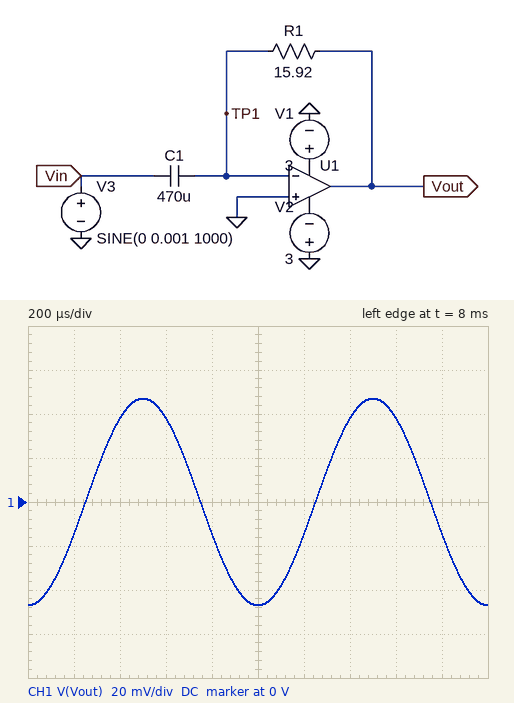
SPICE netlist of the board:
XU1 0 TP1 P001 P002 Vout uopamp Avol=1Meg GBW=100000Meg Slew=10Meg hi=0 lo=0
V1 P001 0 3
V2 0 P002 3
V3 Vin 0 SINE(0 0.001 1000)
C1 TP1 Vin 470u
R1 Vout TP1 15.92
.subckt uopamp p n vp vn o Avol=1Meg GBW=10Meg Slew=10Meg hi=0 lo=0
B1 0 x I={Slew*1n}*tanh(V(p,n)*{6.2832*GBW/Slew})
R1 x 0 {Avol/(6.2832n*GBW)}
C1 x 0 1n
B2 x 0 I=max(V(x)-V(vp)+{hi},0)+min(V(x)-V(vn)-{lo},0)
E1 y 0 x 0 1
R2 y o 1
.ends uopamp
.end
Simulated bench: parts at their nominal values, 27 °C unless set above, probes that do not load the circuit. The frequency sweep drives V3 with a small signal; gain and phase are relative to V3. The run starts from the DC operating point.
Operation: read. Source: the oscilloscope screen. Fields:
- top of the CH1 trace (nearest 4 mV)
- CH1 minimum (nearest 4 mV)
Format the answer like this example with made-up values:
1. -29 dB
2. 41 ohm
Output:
1. 48 mV
2. -48 mV
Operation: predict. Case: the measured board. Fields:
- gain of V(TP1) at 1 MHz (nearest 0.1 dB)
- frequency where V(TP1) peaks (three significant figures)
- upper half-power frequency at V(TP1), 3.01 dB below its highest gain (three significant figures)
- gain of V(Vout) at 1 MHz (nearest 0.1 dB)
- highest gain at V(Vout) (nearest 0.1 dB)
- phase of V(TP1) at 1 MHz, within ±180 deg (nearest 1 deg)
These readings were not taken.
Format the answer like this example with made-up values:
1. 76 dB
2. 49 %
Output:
1. 0 dB
2. 1.42 MHz
3. 1.47 MHz
4. 99.4 dB
5. 119.5 dB
6. 169 deg
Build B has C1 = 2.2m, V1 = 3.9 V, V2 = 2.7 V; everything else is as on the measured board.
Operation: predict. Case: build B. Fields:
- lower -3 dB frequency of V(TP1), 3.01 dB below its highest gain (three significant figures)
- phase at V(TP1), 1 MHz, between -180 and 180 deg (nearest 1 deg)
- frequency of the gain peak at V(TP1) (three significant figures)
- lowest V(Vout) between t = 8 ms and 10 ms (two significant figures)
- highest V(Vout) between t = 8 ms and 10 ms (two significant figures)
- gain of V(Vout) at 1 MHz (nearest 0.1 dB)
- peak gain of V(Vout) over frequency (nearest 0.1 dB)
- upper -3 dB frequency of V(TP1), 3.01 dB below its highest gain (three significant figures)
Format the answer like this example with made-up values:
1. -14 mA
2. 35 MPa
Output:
1. 612 kHz
2. 4 deg
3. 658 kHz
4. -220 mV
5. 220 mV
6. 104.2 dB
7. 119.5 dB
8. 715 kHz
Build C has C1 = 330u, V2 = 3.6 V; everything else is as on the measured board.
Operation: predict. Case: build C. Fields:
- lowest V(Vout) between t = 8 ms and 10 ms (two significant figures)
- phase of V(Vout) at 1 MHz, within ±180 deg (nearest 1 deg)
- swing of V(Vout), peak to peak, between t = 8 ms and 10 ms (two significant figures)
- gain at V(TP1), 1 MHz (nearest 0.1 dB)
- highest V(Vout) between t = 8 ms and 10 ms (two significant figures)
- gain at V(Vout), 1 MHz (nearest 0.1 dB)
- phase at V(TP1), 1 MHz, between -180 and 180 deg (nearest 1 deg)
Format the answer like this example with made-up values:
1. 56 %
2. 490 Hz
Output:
1. -33 mV
2. -93 deg
3. 66 mV
4. -5.3 dB
5. 33 mV
6. 94.1 dB
7. 171 deg
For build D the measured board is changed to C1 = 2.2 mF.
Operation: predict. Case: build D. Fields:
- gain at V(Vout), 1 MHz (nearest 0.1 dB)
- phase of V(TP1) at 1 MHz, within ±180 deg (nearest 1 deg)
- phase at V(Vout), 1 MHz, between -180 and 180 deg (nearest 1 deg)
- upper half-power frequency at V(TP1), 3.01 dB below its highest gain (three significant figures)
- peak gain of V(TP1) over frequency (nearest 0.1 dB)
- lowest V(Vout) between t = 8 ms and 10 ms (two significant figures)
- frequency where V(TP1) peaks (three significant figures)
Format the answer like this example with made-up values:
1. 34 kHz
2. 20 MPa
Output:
1. 104.2 dB
2. 4 deg
3. 100 deg
4. 715 kHz
5. 16.4 dB
6. -220 mV
7. 658 kHz
